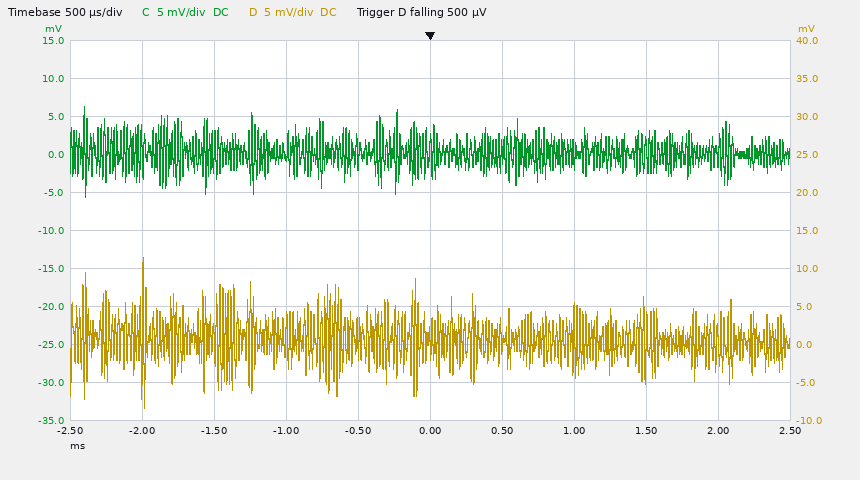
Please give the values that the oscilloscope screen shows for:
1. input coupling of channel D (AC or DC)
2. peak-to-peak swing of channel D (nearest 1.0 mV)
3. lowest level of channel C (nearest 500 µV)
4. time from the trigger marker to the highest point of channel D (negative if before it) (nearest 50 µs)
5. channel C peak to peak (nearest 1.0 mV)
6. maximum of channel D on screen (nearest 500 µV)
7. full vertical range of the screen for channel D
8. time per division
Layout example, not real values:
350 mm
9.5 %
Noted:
DC
20.0 mV
-5.5 mV
-2.00 ms
12.0 mV
11.5 mV
50 mV
500 µs
